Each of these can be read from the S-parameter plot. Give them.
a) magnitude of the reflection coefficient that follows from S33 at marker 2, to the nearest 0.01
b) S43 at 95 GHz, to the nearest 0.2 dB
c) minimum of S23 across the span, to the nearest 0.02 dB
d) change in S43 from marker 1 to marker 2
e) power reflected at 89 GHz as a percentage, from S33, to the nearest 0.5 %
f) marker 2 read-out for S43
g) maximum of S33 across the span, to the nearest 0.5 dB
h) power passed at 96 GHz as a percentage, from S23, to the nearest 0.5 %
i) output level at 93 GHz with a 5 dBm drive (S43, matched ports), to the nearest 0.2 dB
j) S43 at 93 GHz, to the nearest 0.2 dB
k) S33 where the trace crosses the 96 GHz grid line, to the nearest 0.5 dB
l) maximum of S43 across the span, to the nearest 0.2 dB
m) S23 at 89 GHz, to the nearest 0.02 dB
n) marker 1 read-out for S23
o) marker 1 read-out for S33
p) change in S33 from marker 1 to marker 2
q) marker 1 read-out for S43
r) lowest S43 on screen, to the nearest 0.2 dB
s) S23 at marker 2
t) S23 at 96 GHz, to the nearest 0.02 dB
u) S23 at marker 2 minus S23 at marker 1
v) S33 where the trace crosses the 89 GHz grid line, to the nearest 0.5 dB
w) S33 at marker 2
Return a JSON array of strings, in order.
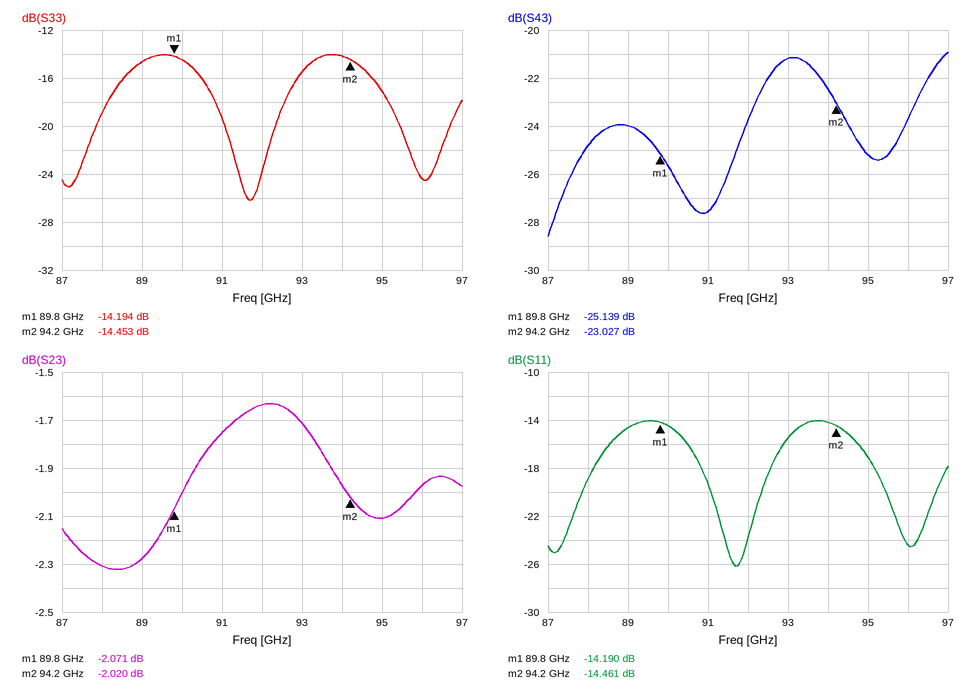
["0.19", "-25.2 dB", "-2.32 dB", "2.112 dB", "3.5 %", "-23.027 dB", "-14.0 dB", "63.5 %", "-16.2 dBm", "-21.2 dB", "-24.5 dB", "-21.0 dB", "-2.28 dB", "-2.071 dB", "-14.194 dB", "-0.259 dB", "-25.139 dB", "-28.6 dB", "-2.020 dB", "-1.98 dB", "0.051 dB", "-14.5 dB", "-14.453 dB"]
